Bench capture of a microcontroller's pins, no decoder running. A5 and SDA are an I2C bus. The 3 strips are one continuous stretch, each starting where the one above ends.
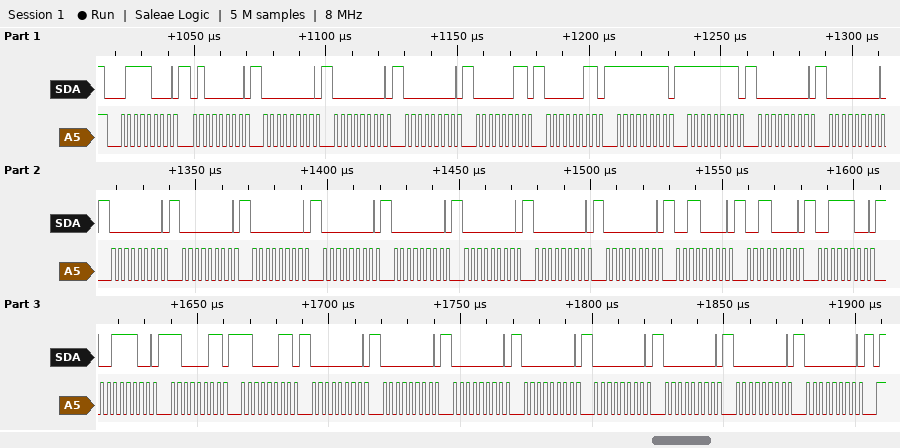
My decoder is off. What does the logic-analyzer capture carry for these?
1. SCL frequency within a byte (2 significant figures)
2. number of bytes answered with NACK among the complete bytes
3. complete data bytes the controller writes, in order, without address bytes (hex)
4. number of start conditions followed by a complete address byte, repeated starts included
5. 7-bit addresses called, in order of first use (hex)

400 kHz
0
40 00 00 00 03 03 FF FF 00 00 00 00 00 00 00 00 00 00 30 30 3C 3C C3 C3 00 00 00 00 00 00 00 00
1
0x3C
